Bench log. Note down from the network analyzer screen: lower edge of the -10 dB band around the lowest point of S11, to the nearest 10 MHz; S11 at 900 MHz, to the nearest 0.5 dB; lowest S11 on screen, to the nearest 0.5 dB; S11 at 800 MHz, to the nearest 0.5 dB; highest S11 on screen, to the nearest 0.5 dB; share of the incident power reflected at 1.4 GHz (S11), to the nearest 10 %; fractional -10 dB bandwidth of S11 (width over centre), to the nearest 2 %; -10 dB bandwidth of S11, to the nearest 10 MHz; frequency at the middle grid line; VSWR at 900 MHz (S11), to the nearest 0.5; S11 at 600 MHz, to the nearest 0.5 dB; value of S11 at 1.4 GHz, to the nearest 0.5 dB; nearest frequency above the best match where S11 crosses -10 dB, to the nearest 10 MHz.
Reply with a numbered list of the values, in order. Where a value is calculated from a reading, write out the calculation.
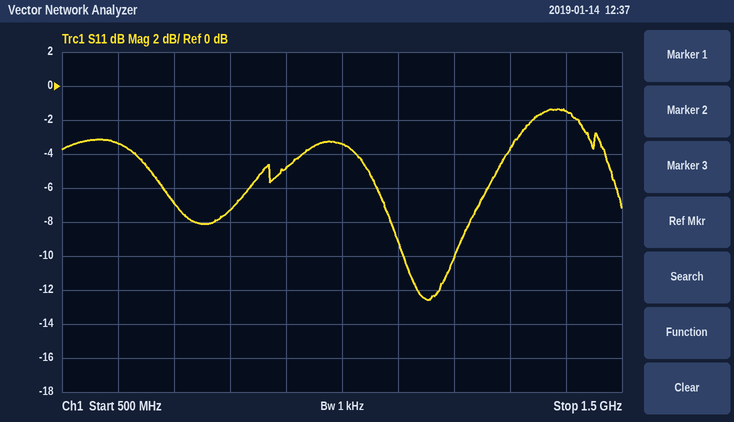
1. 1.11 GHz
2. -5.0 dB
3. -12.5 dB
4. -7.5 dB
5. -1.5 dB
6. 10^(-1.5/10) ≈ 70.8 %, so 70 % to the nearest 10 %
7. 90 MHz / 1.155 GHz ≈ 8 %
8. 1.20 GHz − 1.11 GHz = 90 MHz
9. 1 GHz
10. |Γ| = 10^(-5/20) = 0.5623; VSWR = (1 + 0.5623)/(1 − 0.5623) ≈ 3.57, so 3.5 to the nearest 0.5
11. -3.5 dB
12. -1.5 dB
13. 1.20 GHz
